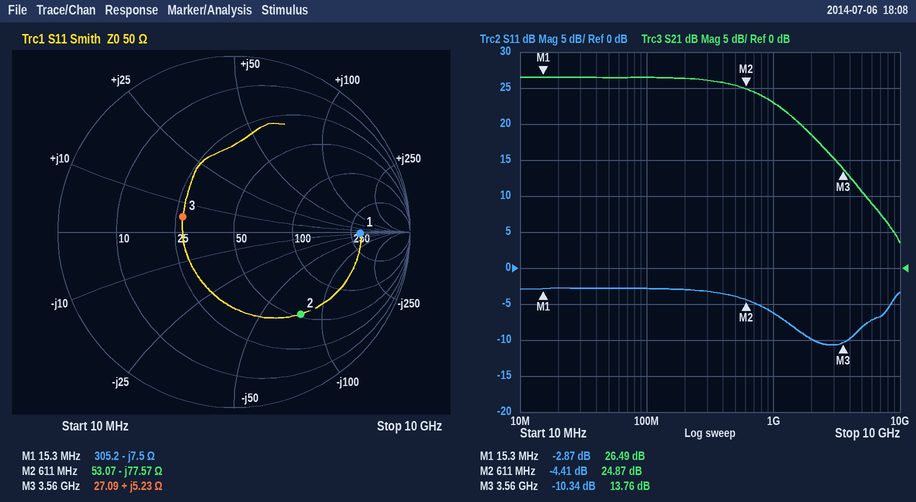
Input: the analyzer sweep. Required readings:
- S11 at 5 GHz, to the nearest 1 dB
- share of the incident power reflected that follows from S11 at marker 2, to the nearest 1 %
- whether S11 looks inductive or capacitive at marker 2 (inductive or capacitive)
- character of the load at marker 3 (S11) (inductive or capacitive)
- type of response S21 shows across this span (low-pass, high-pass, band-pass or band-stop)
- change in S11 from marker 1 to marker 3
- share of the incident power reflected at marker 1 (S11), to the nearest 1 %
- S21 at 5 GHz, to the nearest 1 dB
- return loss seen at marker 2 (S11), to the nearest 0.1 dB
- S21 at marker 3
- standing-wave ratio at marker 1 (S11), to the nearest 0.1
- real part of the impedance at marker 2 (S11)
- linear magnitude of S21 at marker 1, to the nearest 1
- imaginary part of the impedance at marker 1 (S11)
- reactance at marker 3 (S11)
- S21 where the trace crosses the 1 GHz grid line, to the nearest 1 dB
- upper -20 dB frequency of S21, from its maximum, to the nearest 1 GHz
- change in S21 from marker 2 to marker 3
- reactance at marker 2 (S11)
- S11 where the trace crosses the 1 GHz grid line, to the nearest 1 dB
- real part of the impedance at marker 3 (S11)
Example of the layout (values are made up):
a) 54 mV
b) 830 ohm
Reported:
a) -8 dB
b) 36 %
c) capacitive
d) inductive
e) low-pass
f) -7.47 dB
g) 52 %
h) 11 dB
i) 4.4 dB
j) 13.76 dB
k) 6.1
l) 53.07 Ω
m) 21
n) -7.5 Ω
o) +5.23 Ω
p) 23 dB
q) 8 GHz
r) -11.11 dB
s) -77.57 Ω
t) -6 dB
u) 27.09 Ω
